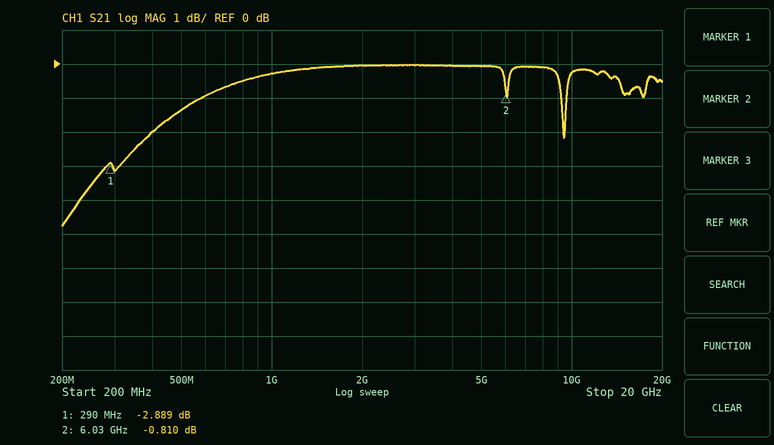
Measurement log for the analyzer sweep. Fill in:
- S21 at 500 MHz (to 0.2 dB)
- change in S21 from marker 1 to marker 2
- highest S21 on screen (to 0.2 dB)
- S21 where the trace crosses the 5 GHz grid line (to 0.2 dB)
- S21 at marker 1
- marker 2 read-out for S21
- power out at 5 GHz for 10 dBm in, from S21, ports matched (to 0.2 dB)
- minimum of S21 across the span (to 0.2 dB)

-1.4 dB
2.079 dB
0.0 dB
0.0 dB
-2.889 dB
-0.810 dB
10.0 dBm
-4.8 dB
